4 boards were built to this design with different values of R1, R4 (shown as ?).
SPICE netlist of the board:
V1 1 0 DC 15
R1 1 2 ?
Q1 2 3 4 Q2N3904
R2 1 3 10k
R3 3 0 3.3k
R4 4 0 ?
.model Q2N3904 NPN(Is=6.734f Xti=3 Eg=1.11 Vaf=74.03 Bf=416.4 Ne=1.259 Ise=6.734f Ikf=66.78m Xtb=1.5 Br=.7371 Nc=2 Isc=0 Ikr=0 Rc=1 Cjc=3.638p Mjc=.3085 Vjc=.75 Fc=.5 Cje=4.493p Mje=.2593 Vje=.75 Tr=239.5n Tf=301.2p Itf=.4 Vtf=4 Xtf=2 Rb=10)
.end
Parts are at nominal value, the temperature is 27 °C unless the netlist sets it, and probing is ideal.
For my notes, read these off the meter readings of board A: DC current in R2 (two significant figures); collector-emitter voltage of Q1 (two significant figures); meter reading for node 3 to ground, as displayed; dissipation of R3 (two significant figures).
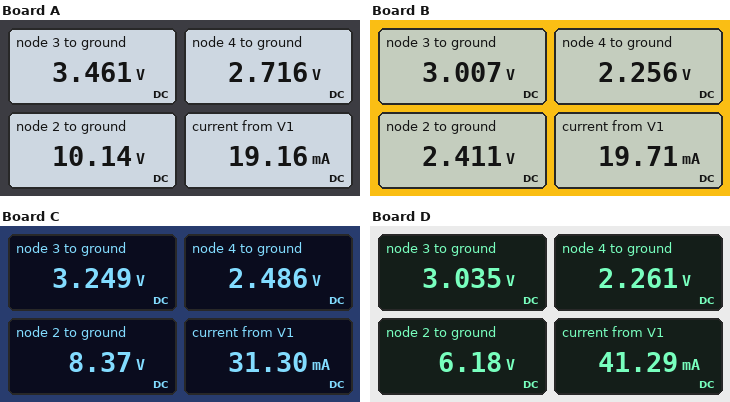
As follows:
1.2 mA
7.4 V
3.461 V
3.6 mW
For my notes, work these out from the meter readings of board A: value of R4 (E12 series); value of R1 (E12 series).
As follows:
150 Ω
270 Ω
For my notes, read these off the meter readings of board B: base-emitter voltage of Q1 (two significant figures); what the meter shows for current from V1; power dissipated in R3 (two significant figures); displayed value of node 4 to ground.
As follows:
750 mV
19.71 mA
2.7 mW
2.256 V
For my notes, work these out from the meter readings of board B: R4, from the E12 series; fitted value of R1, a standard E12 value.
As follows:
120 Ω
680 Ω
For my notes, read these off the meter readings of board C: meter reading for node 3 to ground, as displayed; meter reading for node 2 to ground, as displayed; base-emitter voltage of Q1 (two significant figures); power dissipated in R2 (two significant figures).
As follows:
3.249 V
8.37 V
760 mV
14 mW
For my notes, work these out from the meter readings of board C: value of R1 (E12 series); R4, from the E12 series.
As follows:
220 Ω
82 Ω
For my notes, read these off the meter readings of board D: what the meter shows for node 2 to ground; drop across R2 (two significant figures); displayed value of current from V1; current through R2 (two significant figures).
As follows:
6.18 V
12 V
41.29 mA
1.2 mA
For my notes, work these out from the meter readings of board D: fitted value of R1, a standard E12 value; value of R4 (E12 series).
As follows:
220 Ω
56 Ω
